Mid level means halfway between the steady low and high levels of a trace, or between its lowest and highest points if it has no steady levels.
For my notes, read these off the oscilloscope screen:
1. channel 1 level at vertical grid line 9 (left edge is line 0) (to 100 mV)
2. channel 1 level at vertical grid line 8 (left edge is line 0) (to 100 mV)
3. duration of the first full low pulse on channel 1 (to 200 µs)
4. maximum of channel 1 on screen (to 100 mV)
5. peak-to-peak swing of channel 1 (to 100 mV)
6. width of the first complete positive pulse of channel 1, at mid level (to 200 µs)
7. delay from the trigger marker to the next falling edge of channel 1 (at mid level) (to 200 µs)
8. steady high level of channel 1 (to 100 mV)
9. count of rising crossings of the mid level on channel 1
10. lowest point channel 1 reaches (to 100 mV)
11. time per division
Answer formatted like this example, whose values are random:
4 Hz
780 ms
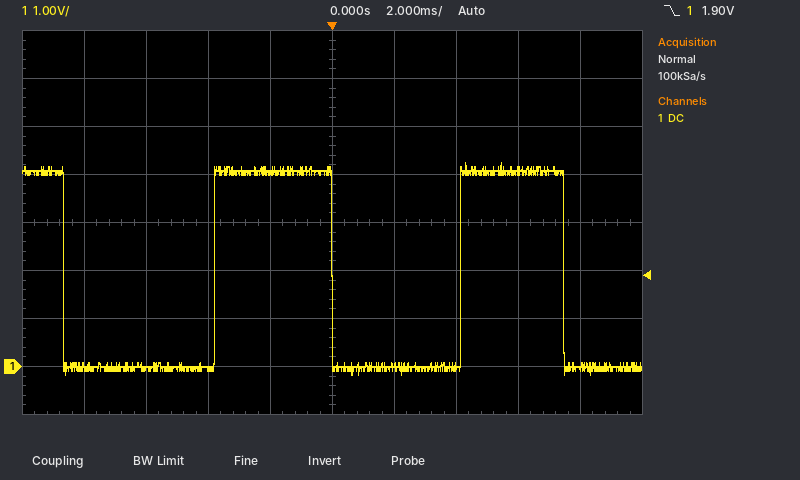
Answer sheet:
0.0 V
4.1 V
4.8 ms
4.2 V
4.4 V
3.8 ms
7.4 ms
4.1 V
2
-200 mV
2 ms
